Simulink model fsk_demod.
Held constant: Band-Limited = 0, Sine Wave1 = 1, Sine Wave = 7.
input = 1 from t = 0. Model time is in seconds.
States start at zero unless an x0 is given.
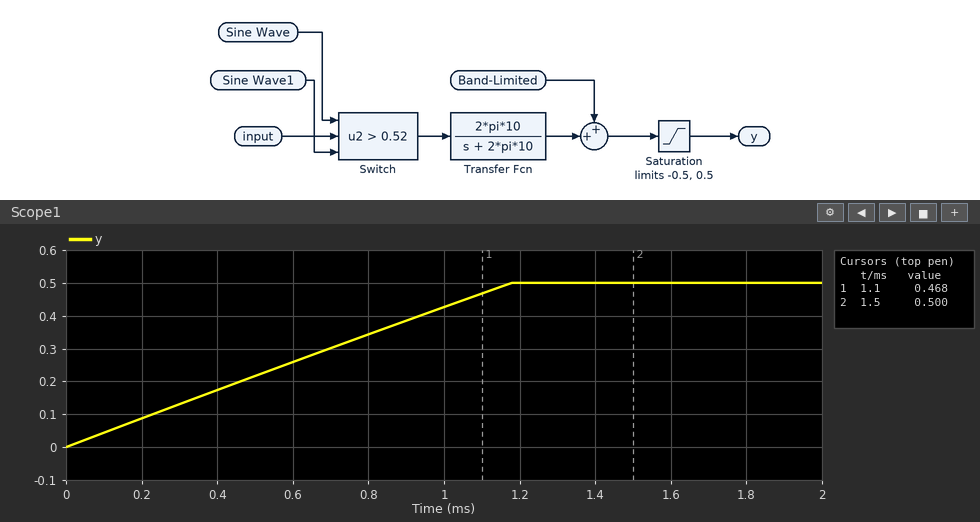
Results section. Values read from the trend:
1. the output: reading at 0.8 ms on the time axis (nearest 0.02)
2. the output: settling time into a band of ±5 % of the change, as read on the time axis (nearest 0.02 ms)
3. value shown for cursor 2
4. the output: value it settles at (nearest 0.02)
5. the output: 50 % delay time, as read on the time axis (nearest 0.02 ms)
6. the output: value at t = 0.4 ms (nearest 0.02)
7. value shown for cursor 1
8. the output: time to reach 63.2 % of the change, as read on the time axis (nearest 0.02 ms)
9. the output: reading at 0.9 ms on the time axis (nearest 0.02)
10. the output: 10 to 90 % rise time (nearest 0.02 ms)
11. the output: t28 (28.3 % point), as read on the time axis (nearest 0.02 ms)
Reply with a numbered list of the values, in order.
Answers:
1. 0.34
2. 1.12 ms
3. 0.500
4. 0.50
5. 0.58 ms
6. 0.18
7. 0.468
8. 0.74 ms
9. 0.38
10. 0.94 ms
11. 0.32 ms
